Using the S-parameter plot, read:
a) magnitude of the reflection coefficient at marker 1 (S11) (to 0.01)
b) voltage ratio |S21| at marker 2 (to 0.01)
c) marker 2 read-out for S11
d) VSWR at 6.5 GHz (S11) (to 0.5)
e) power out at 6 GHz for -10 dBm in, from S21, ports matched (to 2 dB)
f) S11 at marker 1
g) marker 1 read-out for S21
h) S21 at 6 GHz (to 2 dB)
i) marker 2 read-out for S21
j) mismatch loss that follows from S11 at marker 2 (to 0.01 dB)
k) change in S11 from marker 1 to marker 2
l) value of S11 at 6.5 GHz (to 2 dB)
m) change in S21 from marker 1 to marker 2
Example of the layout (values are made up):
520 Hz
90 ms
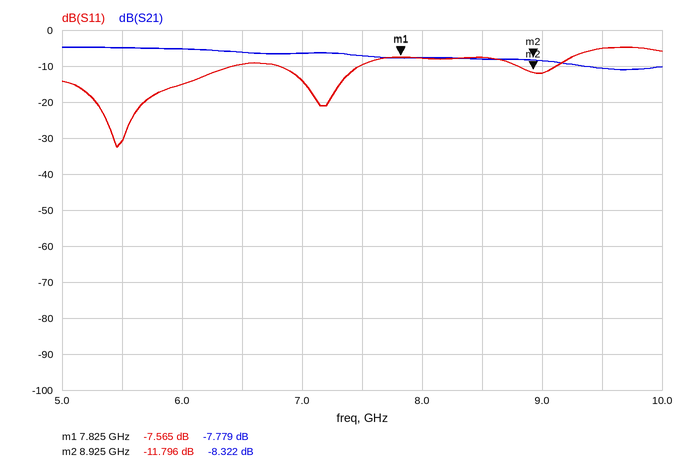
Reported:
0.42
0.38
-11.796 dB
2.0
-16 dBm
-7.565 dB
-7.779 dB
-6 dB
-8.322 dB
0.30 dB
-4.231 dB
-10 dB
-0.543 dB
